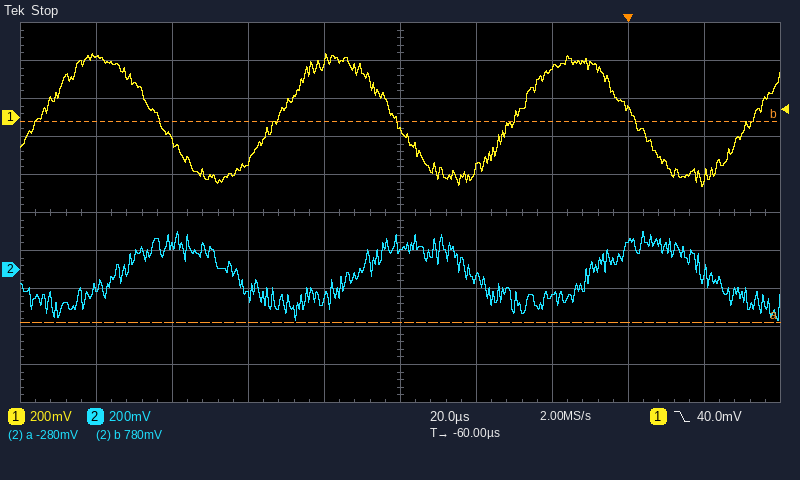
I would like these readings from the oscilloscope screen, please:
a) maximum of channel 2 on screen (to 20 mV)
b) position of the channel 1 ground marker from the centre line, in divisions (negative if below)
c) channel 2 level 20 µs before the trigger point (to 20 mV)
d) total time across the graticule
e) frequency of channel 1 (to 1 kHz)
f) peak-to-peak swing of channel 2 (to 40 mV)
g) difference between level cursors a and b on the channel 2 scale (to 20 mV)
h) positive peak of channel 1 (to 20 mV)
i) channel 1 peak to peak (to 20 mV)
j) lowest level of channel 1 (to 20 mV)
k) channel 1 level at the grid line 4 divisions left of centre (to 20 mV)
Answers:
200 mV
+2.5 div
-140 mV
200 µs
16 kHz
480 mV
1.06 V
340 mV
700 mV
-360 mV
320 mV
